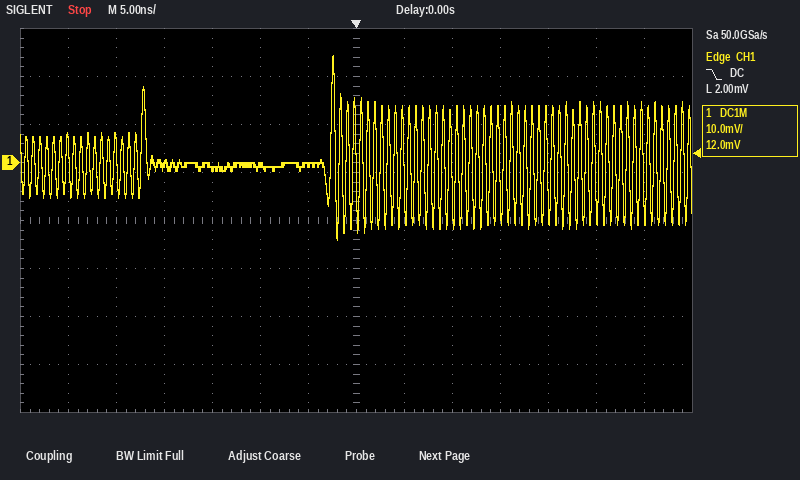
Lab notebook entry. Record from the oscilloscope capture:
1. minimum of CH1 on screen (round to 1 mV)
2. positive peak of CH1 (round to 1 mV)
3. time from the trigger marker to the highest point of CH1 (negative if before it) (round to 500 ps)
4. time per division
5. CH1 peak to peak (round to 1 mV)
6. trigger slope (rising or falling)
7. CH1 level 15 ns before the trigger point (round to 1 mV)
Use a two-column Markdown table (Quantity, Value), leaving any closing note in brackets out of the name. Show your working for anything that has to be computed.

| Quantity | Value |
|---|---|
| minimum of CH1 on screen | -16 mV |
| positive peak of CH1 | 22 mV |
| time from the trigger marker to the highest point of CH1 (negative if before it) | -2.5 ns |
| time per division | 5 ns |
| CH1 peak to peak | 22 mV − (-16 mV) = 38 mV |
| trigger slope | falling |
| CH1 level 15 ns before the trigger point | -1 mV |
